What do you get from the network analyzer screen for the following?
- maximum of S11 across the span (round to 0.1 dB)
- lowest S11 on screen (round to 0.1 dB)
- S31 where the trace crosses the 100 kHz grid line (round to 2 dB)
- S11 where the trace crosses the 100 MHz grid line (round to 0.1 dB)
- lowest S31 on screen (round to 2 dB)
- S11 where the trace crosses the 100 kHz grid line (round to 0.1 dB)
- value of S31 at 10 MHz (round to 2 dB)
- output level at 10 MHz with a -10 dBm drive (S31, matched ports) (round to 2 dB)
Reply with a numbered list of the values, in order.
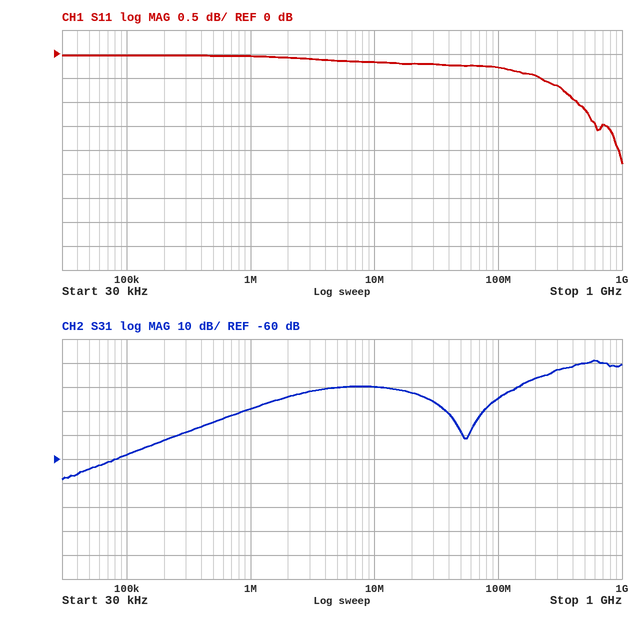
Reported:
1. 0.0 dB
2. -2.3 dB
3. -58 dB
4. -0.3 dB
5. -68 dB
6. 0.0 dB
7. -30 dB
8. -40 dBm
